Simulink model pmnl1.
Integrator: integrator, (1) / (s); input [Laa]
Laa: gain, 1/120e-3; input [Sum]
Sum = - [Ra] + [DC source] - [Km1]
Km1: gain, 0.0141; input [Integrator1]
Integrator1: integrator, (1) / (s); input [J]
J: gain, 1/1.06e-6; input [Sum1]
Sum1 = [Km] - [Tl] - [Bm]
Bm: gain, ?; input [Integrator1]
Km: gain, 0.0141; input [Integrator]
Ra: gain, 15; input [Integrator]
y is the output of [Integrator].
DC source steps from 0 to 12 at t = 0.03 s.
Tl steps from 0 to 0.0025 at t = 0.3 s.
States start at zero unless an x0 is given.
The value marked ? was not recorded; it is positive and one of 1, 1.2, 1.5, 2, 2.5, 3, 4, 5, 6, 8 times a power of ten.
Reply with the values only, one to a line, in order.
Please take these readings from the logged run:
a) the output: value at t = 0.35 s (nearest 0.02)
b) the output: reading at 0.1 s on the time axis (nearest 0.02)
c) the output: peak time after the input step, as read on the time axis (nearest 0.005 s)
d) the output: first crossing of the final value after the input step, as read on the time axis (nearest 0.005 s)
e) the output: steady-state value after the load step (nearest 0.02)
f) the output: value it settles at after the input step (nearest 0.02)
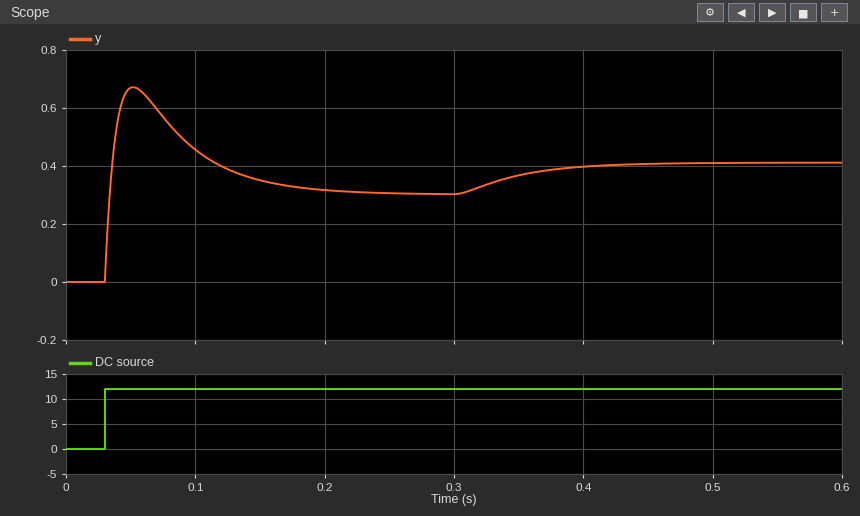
0.36
0.46
0.050 s
0.035 s
0.42
0.30
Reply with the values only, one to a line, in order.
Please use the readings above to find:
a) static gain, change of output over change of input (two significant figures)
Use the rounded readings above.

0.025
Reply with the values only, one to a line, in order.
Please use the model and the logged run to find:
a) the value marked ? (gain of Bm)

8e-06
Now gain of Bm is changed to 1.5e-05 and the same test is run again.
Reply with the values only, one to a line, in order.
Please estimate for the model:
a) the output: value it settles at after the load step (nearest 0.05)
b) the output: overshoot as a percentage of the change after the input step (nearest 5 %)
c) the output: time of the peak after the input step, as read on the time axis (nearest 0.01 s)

0.50
60 %
0.05 s
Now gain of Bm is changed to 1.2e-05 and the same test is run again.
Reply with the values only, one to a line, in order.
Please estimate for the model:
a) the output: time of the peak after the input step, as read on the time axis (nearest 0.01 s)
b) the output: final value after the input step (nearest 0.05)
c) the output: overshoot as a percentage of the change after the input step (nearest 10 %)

0.05 s
0.40
80 %
